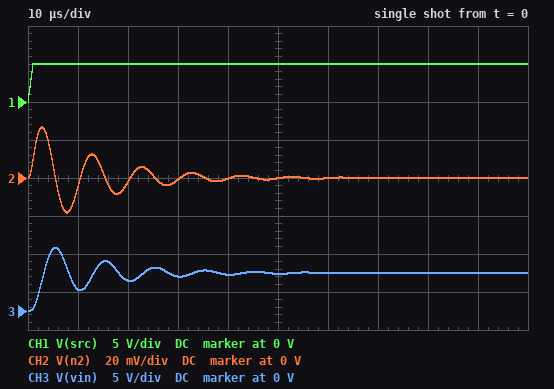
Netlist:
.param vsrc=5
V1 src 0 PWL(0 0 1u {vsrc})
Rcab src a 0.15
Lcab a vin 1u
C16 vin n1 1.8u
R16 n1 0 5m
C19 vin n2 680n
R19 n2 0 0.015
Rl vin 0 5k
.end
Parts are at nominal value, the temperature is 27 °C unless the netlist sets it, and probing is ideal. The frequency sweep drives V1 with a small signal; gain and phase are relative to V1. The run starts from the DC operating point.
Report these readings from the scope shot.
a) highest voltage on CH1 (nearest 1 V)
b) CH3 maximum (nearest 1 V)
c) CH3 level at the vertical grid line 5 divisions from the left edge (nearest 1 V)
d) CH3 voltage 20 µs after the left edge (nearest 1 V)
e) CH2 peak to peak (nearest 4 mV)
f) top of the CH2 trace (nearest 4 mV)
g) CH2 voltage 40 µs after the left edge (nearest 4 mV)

5 V
8 V
5 V
4 V
44 mV
28 mV
0 V
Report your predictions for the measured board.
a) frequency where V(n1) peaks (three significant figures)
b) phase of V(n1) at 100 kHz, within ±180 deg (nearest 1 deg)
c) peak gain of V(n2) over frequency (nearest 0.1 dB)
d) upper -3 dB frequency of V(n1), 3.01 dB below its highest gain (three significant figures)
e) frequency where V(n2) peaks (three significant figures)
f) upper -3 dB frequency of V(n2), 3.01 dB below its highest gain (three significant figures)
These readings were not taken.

101 kHz
5 deg
-31.5 dB
114 kHz
101 kHz
114 kHz
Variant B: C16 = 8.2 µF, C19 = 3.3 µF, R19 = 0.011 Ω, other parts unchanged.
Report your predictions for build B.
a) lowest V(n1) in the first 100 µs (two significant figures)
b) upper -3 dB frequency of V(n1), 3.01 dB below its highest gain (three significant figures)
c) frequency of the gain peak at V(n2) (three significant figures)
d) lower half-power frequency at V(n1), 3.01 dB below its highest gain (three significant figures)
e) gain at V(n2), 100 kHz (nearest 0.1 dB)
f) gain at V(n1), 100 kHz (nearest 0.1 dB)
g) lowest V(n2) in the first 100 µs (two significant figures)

-18 mV
60.7 kHz
46.9 kHz
36.3 kHz
-44.2 dB
-43.2 dB
-16 mV
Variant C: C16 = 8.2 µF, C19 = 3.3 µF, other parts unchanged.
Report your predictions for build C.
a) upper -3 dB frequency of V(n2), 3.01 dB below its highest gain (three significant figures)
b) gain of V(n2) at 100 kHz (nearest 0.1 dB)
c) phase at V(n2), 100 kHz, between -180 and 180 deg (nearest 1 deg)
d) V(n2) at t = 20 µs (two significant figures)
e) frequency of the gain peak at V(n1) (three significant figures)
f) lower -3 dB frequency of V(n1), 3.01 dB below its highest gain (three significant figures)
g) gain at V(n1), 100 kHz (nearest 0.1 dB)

60.7 kHz
-41.5 dB
-73 deg
-11 mV
46.9 kHz
36.3 kHz
-43.2 dB
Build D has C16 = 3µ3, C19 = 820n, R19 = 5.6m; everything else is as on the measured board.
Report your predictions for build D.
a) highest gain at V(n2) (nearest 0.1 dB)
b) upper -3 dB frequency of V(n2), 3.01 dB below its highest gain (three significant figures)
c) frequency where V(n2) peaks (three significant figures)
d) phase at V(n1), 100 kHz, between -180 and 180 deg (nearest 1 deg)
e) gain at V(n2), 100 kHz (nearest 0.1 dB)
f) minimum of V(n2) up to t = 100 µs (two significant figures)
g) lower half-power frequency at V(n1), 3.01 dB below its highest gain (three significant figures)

-42.8 dB
91.6 kHz
78.4 kHz
-58 deg
-48.2 dB
-5.5 mV
67.1 kHz
